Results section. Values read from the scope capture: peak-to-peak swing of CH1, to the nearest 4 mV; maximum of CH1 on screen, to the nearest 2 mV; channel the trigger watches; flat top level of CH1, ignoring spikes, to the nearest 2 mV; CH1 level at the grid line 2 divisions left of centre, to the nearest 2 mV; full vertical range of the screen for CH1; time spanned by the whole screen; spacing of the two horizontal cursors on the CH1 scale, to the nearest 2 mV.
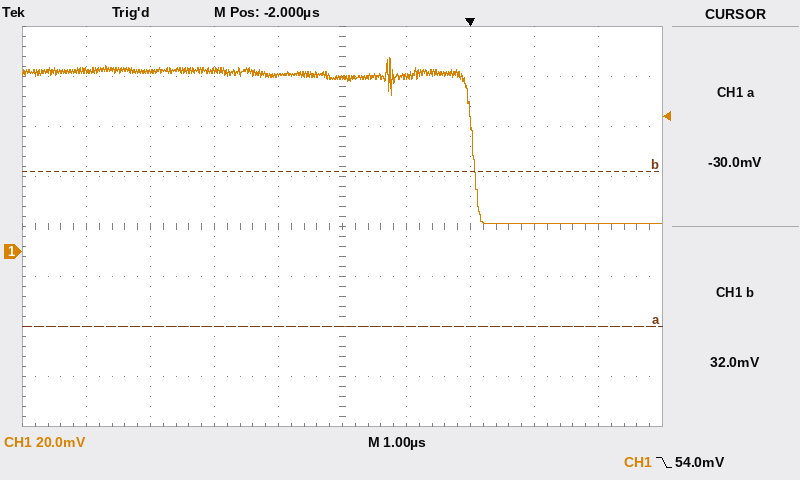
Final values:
68 mV
78 mV
CH1
72 mV
72 mV
160 mV
10 µs
62 mV
